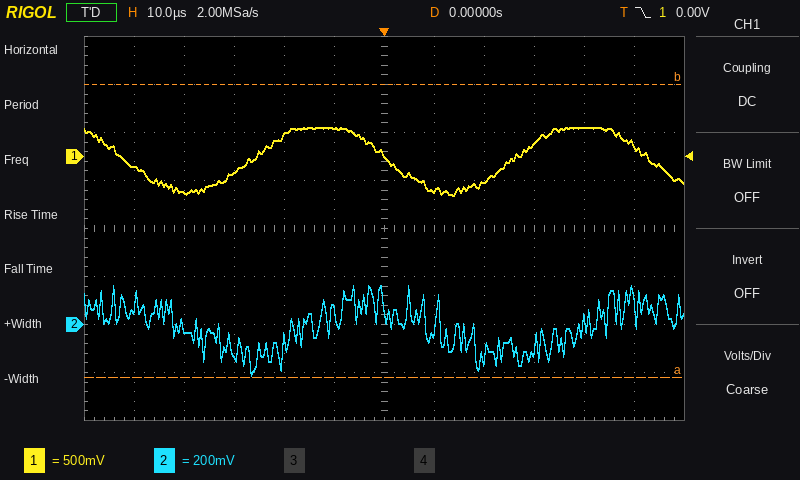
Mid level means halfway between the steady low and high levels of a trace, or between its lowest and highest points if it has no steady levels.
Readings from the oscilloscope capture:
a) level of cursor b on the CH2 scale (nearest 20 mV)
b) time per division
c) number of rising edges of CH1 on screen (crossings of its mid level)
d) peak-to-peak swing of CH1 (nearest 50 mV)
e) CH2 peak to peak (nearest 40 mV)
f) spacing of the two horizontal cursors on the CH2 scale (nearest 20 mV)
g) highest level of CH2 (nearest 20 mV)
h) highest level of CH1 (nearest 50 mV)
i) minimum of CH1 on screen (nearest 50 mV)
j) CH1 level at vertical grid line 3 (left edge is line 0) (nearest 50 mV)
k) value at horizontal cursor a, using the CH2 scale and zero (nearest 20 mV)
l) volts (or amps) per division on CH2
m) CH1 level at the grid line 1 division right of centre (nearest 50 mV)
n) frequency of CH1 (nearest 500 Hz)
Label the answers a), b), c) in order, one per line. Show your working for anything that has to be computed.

a) 1.00 V
b) 10 µs
c) 2
d) 300 mV − (-400 mV) = 700 mV
e) 360 mV
f) 1.22 V
g) 160 mV
h) 300 mV
i) -400 mV
j) -150 mV
k) -220 mV
l) 200 mV
m) -350 mV
n) 19.0 kHz
